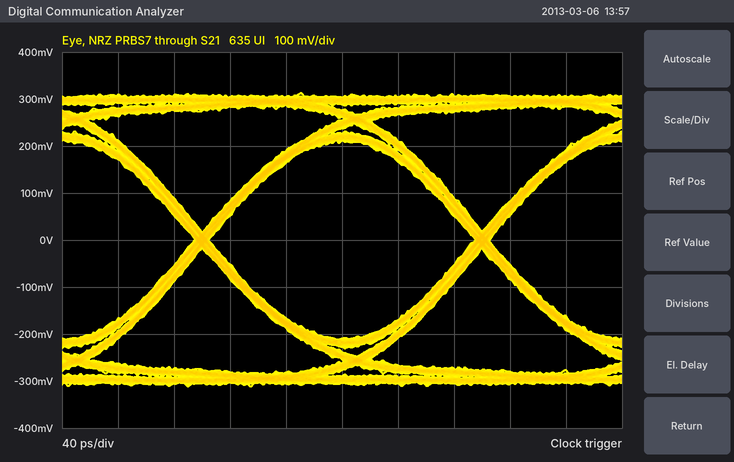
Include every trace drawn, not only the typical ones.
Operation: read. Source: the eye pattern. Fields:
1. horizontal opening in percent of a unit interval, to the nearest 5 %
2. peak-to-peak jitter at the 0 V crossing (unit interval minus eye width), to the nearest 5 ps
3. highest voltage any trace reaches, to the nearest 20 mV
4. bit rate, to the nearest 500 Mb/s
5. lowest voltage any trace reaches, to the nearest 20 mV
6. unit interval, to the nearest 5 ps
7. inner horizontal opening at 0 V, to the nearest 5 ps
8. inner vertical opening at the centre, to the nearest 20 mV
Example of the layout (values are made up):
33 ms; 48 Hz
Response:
95 %; 10 ps; 320 mV; 5.0 Gb/s; -320 mV; 200 ps; 190 ps; 420 mV
